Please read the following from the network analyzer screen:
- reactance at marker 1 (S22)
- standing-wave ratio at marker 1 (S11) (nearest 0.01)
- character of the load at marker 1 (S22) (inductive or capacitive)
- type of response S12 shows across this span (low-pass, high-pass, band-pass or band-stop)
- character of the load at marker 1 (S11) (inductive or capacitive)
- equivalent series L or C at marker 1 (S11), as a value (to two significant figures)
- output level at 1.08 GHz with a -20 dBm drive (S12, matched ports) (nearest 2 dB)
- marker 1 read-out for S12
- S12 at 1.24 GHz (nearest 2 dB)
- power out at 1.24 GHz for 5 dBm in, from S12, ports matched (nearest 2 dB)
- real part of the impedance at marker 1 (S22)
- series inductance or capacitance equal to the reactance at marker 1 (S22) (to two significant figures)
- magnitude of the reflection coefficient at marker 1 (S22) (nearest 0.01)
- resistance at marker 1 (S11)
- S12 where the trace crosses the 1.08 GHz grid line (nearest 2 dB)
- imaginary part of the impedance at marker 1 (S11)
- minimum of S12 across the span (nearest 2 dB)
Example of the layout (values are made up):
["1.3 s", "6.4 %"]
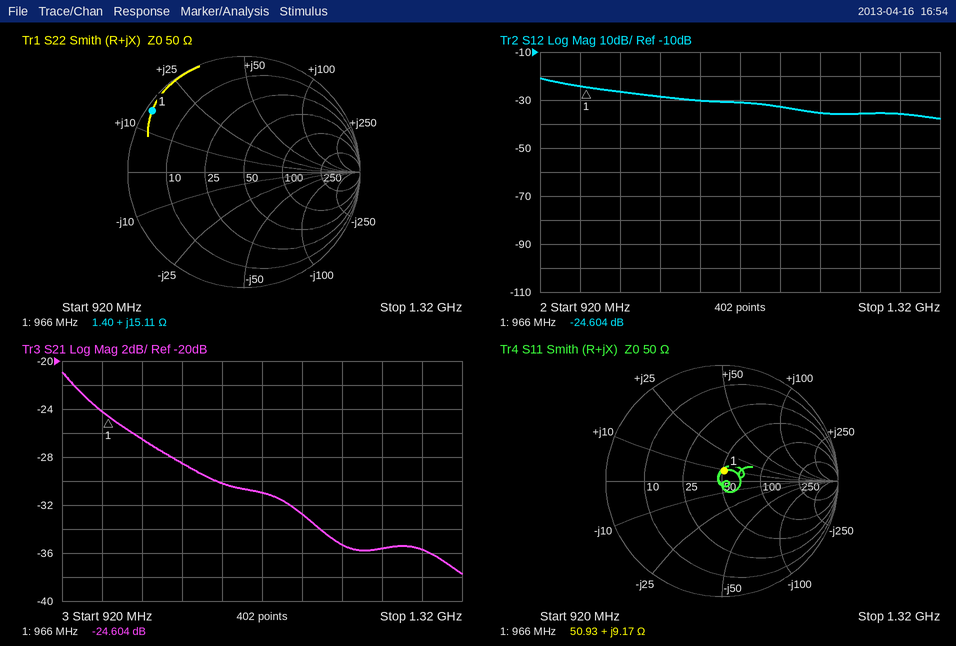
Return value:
["+15.11 Ω", "1.20", "inductive", "low-pass", "inductive", "1.5 nH", "-50 dBm", "-24.604 dB", "-36 dB", "-30 dBm", "1.40 Ω", "2.5 nH", "0.95", "50.93 Ω", "-30 dB", "+9.17 Ω", "-38 dB"]
